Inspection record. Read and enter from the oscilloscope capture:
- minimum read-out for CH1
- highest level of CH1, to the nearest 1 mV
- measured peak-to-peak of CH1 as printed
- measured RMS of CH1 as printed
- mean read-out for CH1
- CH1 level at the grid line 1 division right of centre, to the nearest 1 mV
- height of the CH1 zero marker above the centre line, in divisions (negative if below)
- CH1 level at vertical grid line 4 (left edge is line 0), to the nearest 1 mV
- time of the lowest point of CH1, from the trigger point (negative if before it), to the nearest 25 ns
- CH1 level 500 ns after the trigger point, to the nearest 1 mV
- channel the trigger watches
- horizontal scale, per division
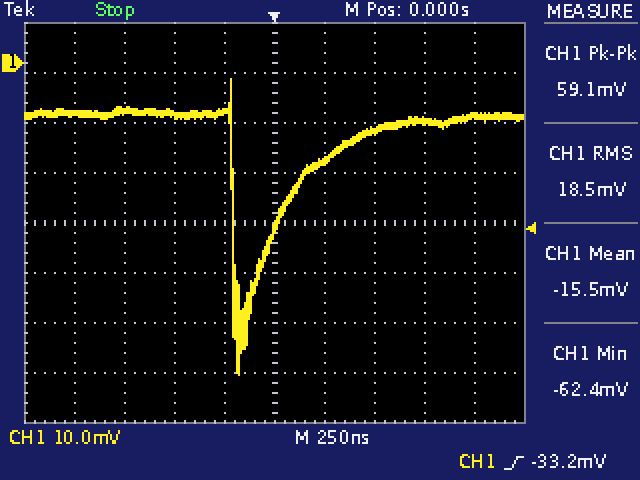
-62.4 mV
-3 mV
59.1 mV
18.5 mV
-15.5 mV
-20 mV
+3.2 div
-10 mV
-175 ns
-14 mV
CH1
250 ns
